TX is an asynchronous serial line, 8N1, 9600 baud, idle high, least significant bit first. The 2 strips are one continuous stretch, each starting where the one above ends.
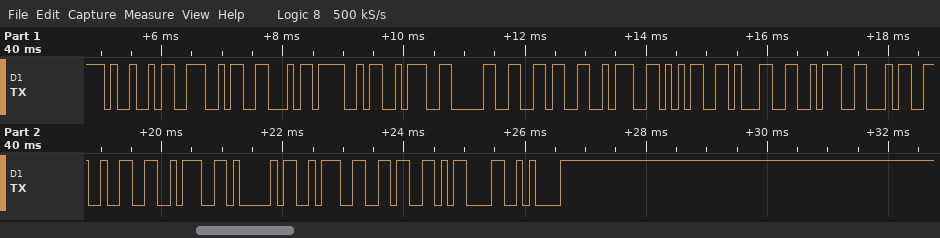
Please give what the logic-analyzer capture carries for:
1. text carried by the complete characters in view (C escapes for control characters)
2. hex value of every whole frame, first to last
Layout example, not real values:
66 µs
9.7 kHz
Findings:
"INFO:06:51:42:A:6\r\n"
0x49 0x4E 0x46 0x4F 0x3A 0x30 0x36 0x3A 0x35 0x31 0x3A 0x34 0x32 0x3A 0x41 0x3A 0x36 0x0D 0x0A
